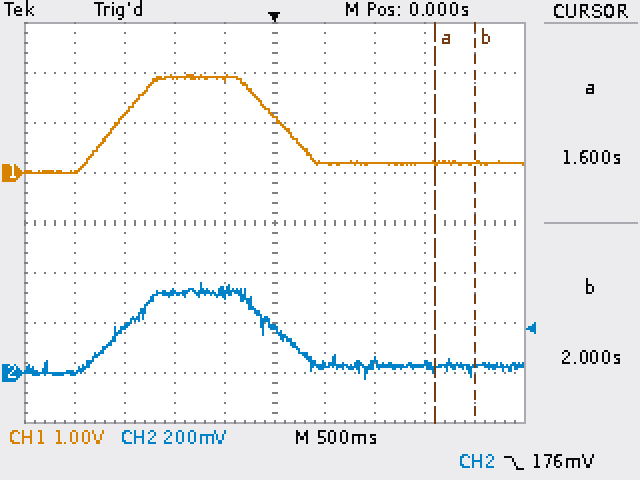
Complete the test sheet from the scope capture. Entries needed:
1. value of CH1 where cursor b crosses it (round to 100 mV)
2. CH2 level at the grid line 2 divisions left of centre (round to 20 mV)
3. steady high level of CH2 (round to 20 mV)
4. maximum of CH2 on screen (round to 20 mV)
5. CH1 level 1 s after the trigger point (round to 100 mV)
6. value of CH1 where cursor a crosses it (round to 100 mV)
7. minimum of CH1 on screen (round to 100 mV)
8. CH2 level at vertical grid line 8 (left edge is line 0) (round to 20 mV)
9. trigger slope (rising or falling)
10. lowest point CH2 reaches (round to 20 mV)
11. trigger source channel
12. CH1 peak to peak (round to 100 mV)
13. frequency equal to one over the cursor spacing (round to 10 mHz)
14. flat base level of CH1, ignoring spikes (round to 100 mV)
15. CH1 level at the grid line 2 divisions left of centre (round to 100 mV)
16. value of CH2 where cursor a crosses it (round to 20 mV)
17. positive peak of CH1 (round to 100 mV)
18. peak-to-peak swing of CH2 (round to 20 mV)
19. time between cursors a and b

200 mV
320 mV
320 mV
360 mV
200 mV
200 mV
0.0 V
40 mV
falling
-20 mV
CH2
2.0 V
2.50 Hz
200 mV
1.9 V
20 mV
2.0 V
380 mV
400 ms
